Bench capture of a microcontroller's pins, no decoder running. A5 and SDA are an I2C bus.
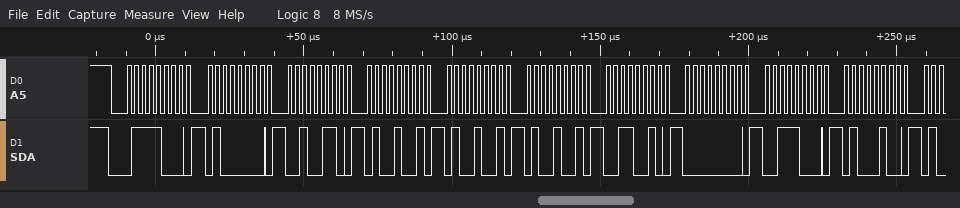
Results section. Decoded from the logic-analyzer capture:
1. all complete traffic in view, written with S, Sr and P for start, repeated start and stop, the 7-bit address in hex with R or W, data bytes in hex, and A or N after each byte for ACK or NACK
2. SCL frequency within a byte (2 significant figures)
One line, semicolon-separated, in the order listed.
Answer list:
S 3CW A 40 A 26 A 49 A 49 A 49 A 32 A 00 A 38 A 44 A; 400 kHz
